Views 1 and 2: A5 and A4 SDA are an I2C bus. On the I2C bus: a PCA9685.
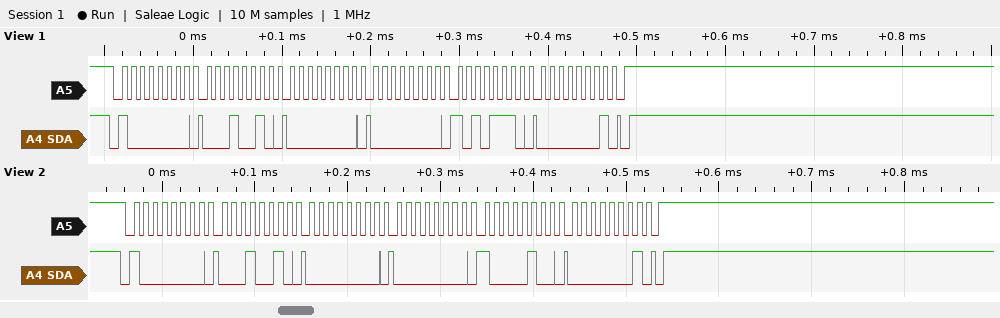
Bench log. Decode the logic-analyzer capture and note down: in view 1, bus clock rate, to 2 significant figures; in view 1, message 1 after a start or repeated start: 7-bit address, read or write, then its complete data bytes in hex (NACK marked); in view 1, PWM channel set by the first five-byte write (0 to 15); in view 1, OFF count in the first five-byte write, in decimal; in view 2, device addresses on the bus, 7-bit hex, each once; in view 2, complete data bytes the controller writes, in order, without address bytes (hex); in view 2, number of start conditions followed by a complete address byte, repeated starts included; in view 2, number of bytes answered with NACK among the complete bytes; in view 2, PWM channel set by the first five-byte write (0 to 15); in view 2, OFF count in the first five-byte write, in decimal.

100 kHz
0x40 write: 12 00 00 AE 01
3
430
0x40
12 00 00 84 01
1
0
3
388
